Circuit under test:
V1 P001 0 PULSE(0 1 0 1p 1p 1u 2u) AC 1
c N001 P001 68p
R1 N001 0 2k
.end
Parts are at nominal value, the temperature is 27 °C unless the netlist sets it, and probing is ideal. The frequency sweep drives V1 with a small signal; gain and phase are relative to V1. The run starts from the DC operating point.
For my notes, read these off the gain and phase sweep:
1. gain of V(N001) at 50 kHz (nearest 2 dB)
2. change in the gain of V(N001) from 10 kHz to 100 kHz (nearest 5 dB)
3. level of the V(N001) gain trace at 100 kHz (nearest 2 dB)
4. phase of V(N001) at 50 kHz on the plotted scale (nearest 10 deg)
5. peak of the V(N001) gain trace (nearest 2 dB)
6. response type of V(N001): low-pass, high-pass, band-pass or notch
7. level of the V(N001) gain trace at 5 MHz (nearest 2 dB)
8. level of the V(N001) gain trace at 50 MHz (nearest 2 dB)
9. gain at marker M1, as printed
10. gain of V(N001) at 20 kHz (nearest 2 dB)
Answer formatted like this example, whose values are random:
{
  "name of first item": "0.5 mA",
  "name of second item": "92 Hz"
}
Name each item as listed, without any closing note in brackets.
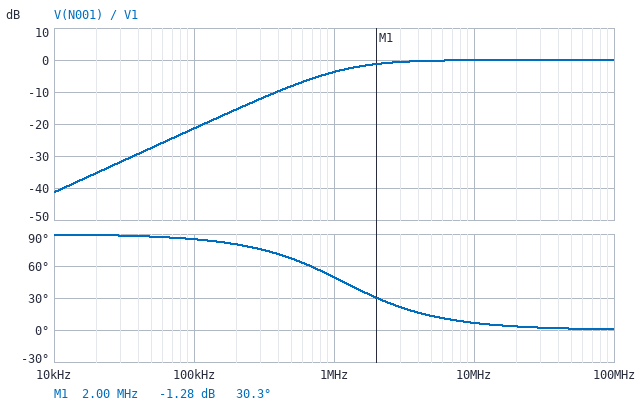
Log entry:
{
  "gain of V(N001) at 50 kHz": "-28 dB",
  "change in the gain of V(N001) from 10 kHz to 100 kHz": "20 dB",
  "level of the V(N001) gain trace at 100 kHz": "-22 dB",
  "phase of V(N001) at 50 kHz on the plotted scale": "90 deg",
  "peak of the V(N001) gain trace": "0 dB",
  "response type of V(N001): low-pass, high-pass, band-pass or notch": "high-pass",
  "level of the V(N001) gain trace at 5 MHz": "0 dB",
  "level of the V(N001) gain trace at 50 MHz": "0 dB",
  "gain at marker M1, as printed": "-1.28 dB",
  "gain of V(N001) at 20 kHz": "-36 dB"
}
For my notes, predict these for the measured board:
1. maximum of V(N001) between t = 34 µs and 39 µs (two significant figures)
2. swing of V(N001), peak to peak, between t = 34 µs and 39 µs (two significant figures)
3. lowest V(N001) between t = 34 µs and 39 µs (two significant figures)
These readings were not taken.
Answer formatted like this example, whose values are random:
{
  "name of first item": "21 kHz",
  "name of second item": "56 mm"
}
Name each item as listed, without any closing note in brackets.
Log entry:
{
  "maximum of V(N001) between t = 34 µs and 39 µs": "1.0 V",
  "swing of V(N001), peak to peak, between t = 34 µs and 39 µs": "2.0 V",
  "lowest V(N001) between t = 34 µs and 39 µs": "-1.0 V"
}
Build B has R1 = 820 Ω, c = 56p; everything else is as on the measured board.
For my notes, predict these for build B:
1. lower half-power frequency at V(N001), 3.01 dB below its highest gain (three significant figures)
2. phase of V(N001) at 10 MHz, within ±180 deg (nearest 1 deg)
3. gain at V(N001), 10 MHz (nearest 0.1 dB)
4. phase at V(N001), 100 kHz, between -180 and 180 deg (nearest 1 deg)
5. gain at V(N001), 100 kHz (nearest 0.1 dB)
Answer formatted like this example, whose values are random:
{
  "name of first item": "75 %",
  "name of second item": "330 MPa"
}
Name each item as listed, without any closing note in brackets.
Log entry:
{
  "lower half-power frequency at V(N001), 3.01 dB below its highest gain": "3.47 MHz",
  "phase of V(N001) at 10 MHz, within ±180 deg": "19 deg",
  "gain at V(N001), 10 MHz": "-0.5 dB",
  "phase at V(N001), 100 kHz, between -180 and 180 deg": "88 deg",
  "gain at V(N001), 100 kHz": "-30.8 dB"
}
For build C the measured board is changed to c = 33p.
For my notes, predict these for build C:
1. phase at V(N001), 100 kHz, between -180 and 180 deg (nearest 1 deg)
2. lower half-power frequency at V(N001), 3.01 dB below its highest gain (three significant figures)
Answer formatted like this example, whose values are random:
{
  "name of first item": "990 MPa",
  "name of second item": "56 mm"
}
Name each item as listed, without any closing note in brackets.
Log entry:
{
  "phase at V(N001), 100 kHz, between -180 and 180 deg": "88 deg",
  "lower half-power frequency at V(N001), 3.01 dB below its highest gain": "2.41 MHz"
}
